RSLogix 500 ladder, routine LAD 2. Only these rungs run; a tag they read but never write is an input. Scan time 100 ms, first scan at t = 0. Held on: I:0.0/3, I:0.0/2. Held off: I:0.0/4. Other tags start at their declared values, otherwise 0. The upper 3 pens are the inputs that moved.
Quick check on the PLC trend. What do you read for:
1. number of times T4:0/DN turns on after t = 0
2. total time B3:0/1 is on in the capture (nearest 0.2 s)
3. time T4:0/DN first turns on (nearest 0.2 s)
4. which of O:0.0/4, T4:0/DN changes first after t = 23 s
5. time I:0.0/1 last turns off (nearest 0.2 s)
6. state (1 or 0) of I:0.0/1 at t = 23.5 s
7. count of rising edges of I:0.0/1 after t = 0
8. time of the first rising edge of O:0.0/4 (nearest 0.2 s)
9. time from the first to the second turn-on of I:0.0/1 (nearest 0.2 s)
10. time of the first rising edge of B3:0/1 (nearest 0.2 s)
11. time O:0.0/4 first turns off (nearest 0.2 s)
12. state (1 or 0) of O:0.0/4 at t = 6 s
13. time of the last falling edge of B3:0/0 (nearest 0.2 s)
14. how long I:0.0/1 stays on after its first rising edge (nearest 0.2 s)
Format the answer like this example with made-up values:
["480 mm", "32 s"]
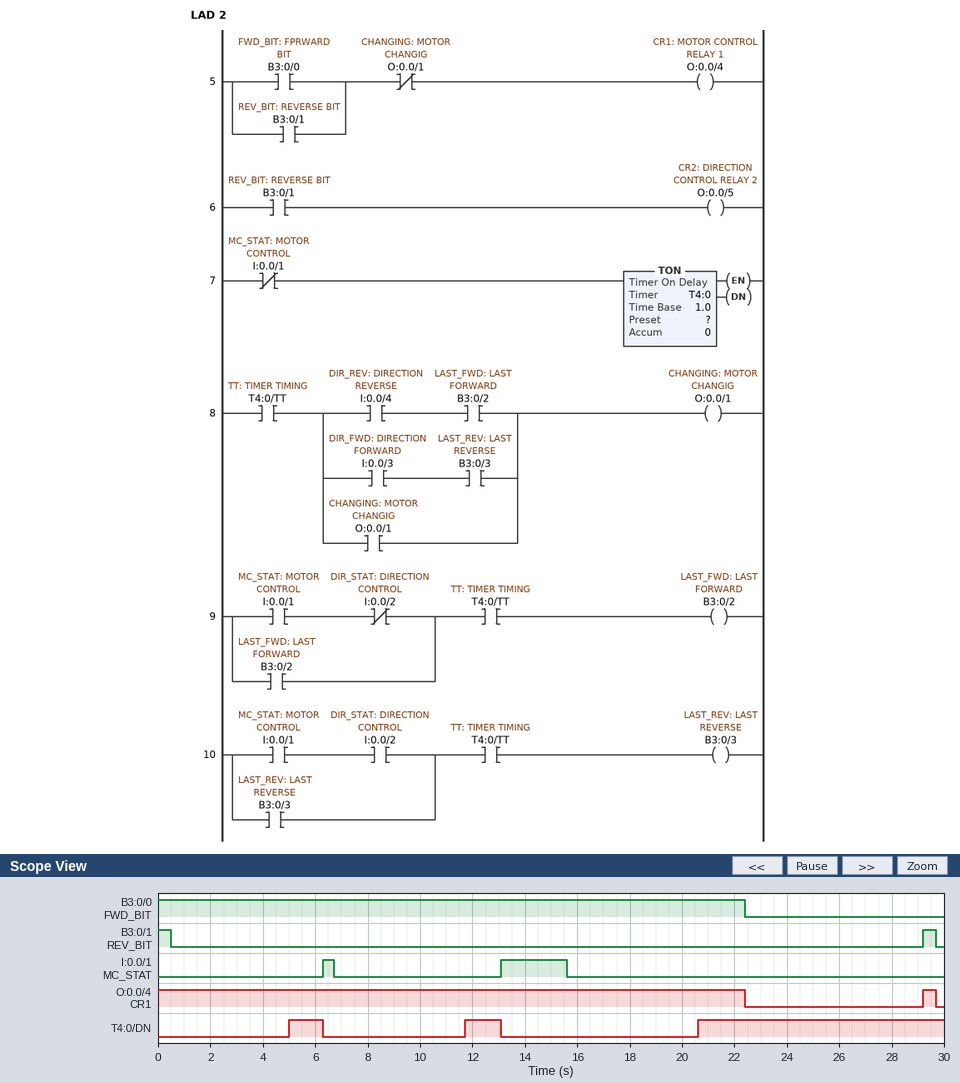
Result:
["3", "1.0 s", "5.0 s", "O:0.0/4", "15.6 s", "0", "2", "29.2 s", "6.8 s", "29.2 s", "22.4 s", "1", "22.4 s", "0.4 s"]
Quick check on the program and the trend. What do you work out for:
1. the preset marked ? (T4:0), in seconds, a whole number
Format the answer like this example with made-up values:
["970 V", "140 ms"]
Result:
["5 s"]
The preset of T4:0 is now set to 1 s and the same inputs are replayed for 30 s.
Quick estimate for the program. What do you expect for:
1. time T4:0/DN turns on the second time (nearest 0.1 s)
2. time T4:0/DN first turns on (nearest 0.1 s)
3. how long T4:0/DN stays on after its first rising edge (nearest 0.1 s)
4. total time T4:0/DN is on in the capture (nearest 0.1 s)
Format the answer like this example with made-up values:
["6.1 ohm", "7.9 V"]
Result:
["7.7 s", "1.0 s", "5.3 s", "24.1 s"]
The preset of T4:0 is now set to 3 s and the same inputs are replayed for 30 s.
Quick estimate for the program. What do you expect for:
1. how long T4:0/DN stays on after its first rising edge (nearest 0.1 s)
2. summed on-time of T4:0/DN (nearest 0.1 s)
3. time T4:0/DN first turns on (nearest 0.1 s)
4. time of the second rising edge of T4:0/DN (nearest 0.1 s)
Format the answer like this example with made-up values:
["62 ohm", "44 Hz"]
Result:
["3.3 s", "18.1 s", "3.0 s", "9.7 s"]
